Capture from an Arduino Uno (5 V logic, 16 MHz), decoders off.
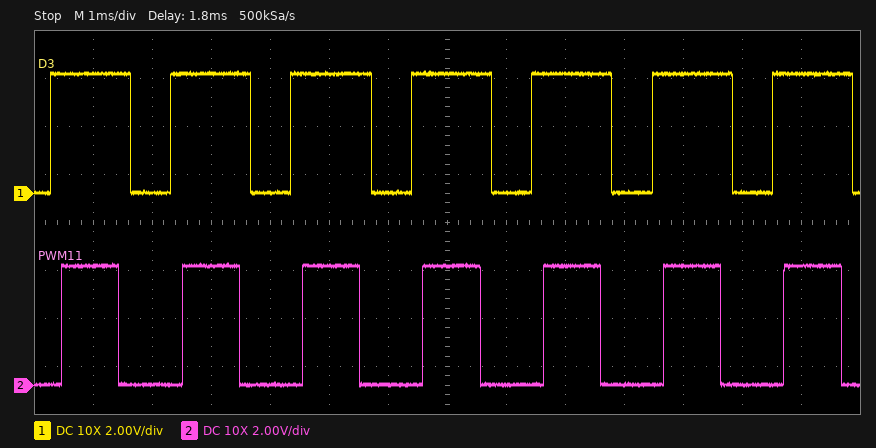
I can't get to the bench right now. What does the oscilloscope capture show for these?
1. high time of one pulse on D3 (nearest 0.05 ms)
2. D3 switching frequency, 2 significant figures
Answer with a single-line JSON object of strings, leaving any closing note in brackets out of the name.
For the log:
{"high time of one pulse on D3": "1.35 ms", "D3 switching frequency, 2 significant figures": "490 Hz"}
